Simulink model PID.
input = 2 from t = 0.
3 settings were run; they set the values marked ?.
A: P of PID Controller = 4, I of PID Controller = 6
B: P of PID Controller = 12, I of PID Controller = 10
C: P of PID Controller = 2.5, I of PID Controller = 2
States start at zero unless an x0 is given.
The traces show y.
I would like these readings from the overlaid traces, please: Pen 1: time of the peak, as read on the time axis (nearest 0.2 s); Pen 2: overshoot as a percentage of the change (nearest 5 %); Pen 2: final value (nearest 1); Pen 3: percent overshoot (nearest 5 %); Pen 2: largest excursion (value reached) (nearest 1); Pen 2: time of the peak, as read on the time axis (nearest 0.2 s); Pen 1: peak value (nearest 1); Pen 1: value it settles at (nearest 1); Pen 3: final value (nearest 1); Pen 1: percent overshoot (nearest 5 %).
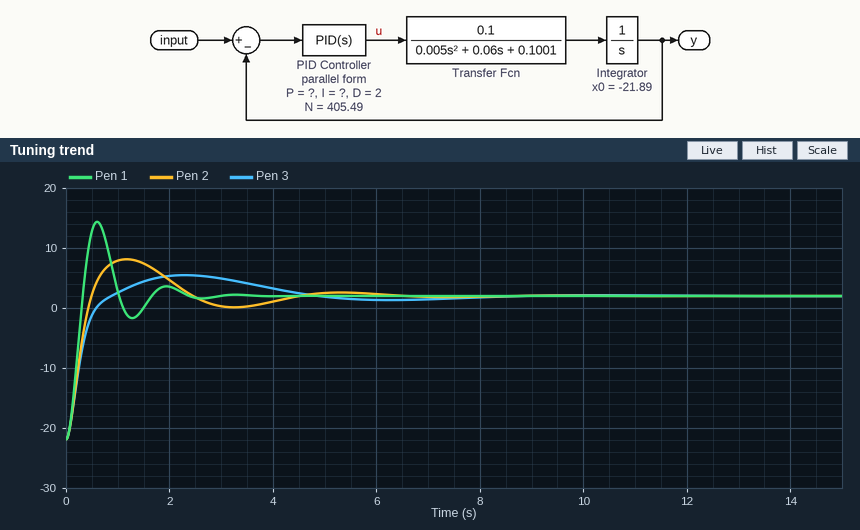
0.6 s
25 %
2
15 %
8
1.2 s
14
2
2
50 %
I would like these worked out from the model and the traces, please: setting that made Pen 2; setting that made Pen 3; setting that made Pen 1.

A
C
B
